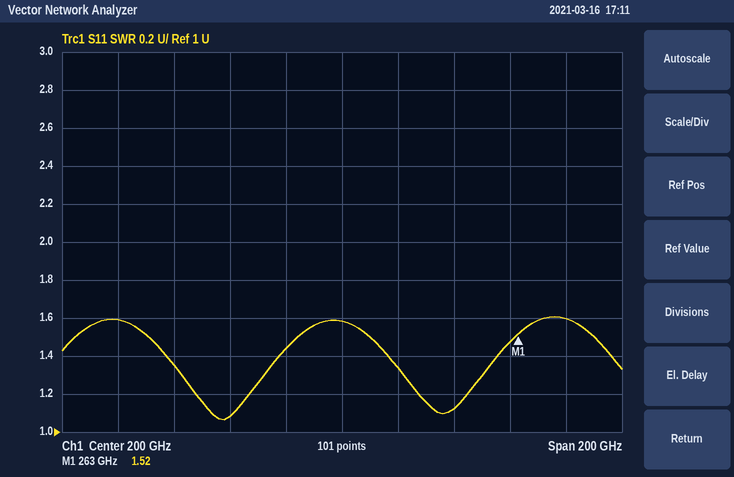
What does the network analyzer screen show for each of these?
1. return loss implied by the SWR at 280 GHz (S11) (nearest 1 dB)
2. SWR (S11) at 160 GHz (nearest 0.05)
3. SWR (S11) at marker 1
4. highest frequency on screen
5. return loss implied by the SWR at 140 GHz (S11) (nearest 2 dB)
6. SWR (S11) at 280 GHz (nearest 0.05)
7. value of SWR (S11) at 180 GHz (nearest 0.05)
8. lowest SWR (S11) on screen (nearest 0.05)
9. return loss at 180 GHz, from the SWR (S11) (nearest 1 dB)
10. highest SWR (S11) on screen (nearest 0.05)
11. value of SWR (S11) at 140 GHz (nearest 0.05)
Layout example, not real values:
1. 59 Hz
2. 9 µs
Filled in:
1. 13 dB
2. 1.10
3. 1.52
4. 300 GHz
5. 16 dB
6. 1.60
7. 1.45
8. 1.05
9. 15 dB
10. 1.60
11. 1.35
